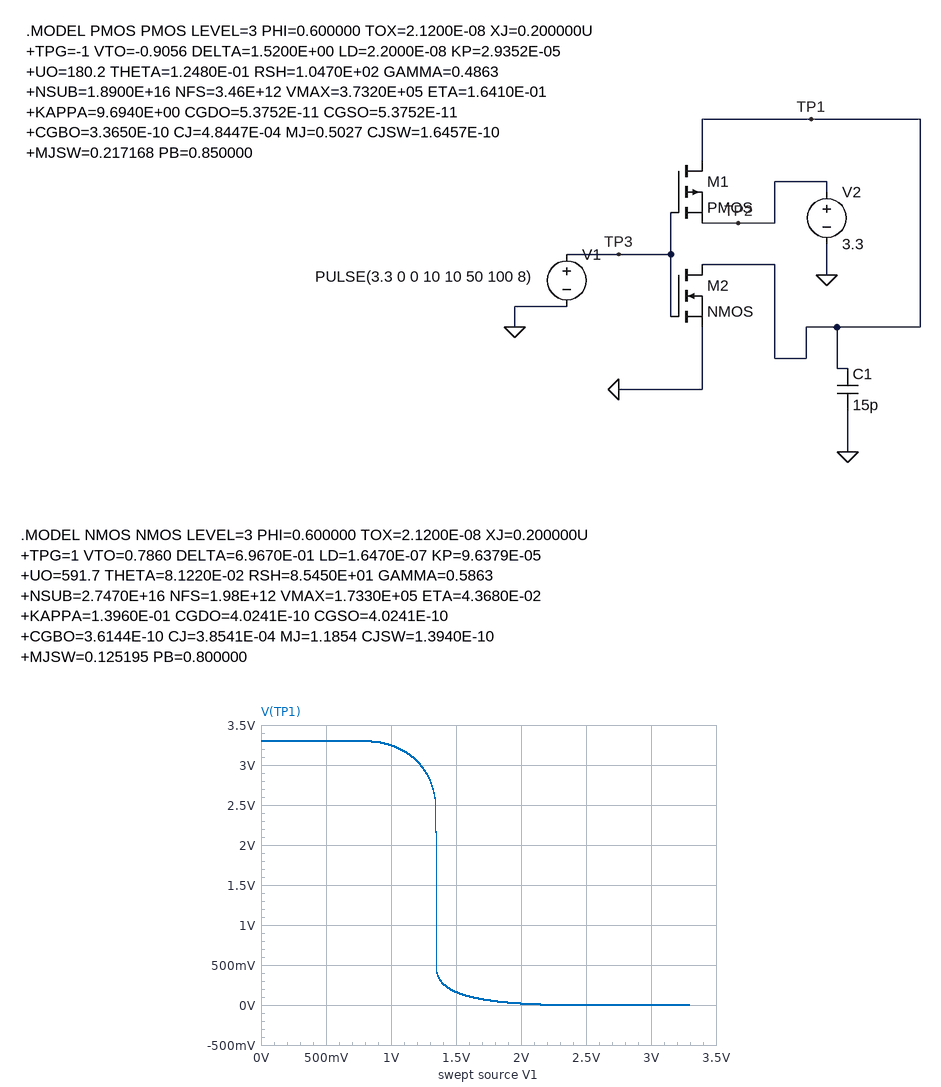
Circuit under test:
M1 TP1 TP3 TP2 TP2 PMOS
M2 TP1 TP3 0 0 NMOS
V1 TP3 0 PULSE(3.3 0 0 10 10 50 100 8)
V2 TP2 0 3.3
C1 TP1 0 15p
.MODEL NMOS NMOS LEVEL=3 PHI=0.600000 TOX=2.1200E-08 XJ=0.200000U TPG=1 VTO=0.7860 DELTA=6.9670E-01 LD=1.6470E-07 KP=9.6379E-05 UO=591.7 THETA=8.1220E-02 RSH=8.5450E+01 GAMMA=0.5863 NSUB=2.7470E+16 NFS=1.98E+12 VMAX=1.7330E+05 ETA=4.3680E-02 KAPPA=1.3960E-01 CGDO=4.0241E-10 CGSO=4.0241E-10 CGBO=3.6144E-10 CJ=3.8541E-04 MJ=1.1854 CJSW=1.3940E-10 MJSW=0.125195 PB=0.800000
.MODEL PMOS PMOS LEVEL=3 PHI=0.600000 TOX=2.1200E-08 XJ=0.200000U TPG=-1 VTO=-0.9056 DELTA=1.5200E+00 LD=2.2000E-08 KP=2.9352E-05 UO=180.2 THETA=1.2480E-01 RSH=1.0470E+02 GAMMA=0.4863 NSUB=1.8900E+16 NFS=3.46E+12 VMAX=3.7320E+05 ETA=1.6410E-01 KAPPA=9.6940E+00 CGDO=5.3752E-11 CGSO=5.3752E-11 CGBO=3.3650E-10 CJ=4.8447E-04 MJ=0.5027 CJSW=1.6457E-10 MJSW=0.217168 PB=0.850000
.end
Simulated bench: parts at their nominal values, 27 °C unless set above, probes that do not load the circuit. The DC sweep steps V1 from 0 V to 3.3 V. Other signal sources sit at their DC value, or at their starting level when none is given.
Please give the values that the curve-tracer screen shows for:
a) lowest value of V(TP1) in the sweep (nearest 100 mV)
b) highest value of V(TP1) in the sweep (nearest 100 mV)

0 V
3.3 V
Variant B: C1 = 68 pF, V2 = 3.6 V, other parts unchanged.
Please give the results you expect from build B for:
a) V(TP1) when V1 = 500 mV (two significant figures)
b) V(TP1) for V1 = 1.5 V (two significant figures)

3.6 V
340 mV
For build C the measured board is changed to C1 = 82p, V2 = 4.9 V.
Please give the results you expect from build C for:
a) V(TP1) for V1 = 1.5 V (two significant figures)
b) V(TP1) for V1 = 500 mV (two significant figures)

4.5 V
4.9 V
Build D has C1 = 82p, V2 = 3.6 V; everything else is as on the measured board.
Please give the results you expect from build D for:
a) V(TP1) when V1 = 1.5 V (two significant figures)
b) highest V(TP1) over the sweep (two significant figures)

340 mV
3.6 V
